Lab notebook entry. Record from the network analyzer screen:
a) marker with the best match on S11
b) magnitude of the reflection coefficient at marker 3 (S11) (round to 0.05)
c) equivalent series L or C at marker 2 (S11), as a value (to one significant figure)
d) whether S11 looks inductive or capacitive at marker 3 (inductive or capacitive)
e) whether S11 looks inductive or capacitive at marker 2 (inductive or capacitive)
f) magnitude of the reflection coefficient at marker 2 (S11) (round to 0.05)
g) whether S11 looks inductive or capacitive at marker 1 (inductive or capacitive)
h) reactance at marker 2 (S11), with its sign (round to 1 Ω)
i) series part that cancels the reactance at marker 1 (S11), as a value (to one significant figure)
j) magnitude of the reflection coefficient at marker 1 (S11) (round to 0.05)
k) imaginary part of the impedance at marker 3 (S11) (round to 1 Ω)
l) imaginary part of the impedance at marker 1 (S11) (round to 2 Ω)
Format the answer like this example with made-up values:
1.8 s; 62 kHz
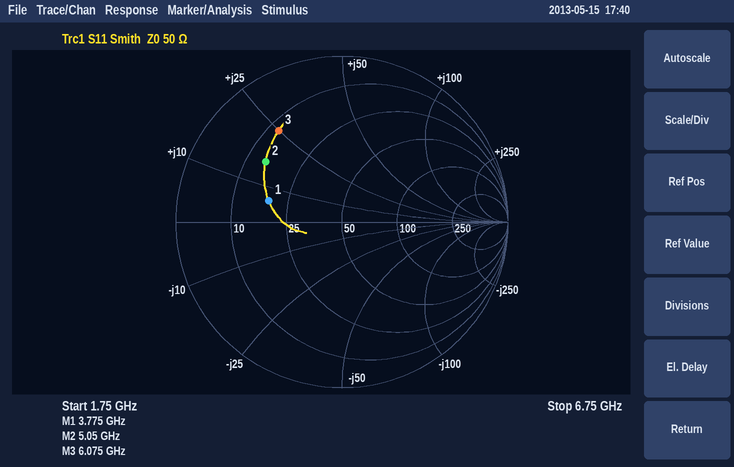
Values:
marker 1; 0.65; 500 pH; inductive; inductive; 0.60; inductive; +16 Ω; 7 pF; 0.45; +25 Ω; +6 Ω
